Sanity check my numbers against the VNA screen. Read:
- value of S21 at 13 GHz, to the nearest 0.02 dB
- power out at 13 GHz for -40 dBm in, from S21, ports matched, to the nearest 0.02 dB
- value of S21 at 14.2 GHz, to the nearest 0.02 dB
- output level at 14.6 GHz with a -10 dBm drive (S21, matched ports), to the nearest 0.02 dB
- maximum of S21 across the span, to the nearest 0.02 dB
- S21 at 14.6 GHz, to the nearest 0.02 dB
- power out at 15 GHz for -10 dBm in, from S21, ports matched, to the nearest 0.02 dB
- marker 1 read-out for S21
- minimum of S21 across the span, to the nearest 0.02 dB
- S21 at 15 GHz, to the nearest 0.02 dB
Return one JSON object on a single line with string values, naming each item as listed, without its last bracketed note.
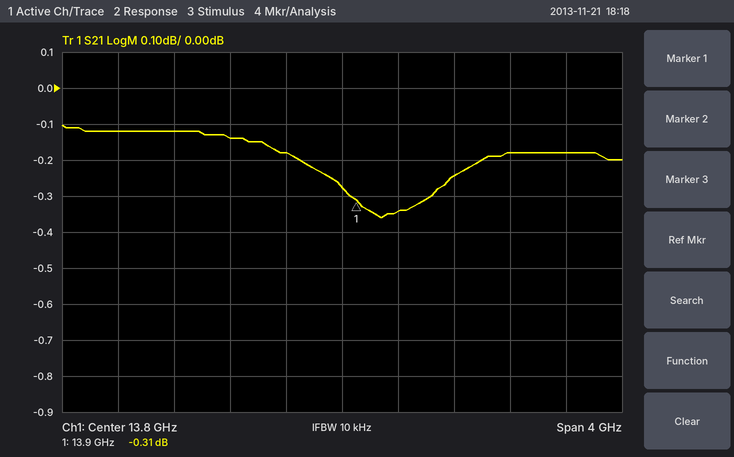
{"value of S21 at 13 GHz, to the nearest 0.02 dB": "-0.14 dB", "power out at 13 GHz for -40 dBm in, from S21, ports matched, to the nearest 0.02 dB": "-40.14 dBm", "value of S21 at 14.2 GHz, to the nearest 0.02 dB": "-0.34 dB", "output level at 14.6 GHz with a -10 dBm drive (S21, matched ports), to the nearest 0.02 dB": "-10.24 dBm", "maximum of S21 across the span, to the nearest 0.02 dB": "-0.10 dB", "S21 at 14.6 GHz, to the nearest 0.02 dB": "-0.24 dB", "power out at 15 GHz for -10 dBm in, from S21, ports matched, to the nearest 0.02 dB": "-10.18 dBm", "marker 1 read-out for S21": "-0.31 dB", "minimum of S21 across the span, to the nearest 0.02 dB": "-0.36 dB", "S21 at 15 GHz, to the nearest 0.02 dB": "-0.18 dB"}
